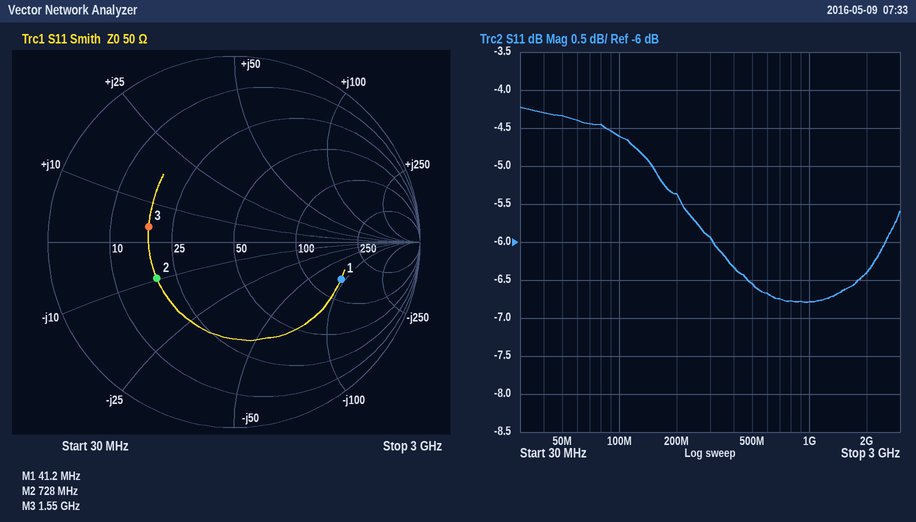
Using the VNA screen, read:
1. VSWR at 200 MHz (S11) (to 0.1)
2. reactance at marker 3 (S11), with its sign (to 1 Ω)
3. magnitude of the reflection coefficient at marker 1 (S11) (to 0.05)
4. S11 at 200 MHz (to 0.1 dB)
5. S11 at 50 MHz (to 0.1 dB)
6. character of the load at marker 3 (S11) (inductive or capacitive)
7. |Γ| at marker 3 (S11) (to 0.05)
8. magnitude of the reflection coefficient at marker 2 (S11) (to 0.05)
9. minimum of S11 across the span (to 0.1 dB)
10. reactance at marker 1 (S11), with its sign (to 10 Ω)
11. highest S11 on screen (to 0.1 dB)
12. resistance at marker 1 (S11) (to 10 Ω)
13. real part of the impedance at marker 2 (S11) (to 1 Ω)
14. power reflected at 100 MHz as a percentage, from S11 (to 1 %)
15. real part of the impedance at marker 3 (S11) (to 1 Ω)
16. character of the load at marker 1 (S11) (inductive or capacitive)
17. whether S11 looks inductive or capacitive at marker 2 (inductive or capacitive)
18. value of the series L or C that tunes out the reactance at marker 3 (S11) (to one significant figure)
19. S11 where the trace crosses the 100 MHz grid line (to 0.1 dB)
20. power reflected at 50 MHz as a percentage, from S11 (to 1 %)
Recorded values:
3.3
+4 Ω
0.60
-5.4 dB
-4.3 dB
inductive
0.45
0.45
-6.8 dB
-90 Ω
-4.2 dB
140 Ω
19 Ω
35 %
18 Ω
capacitive
capacitive
30 pF
-4.6 dB
37 %
